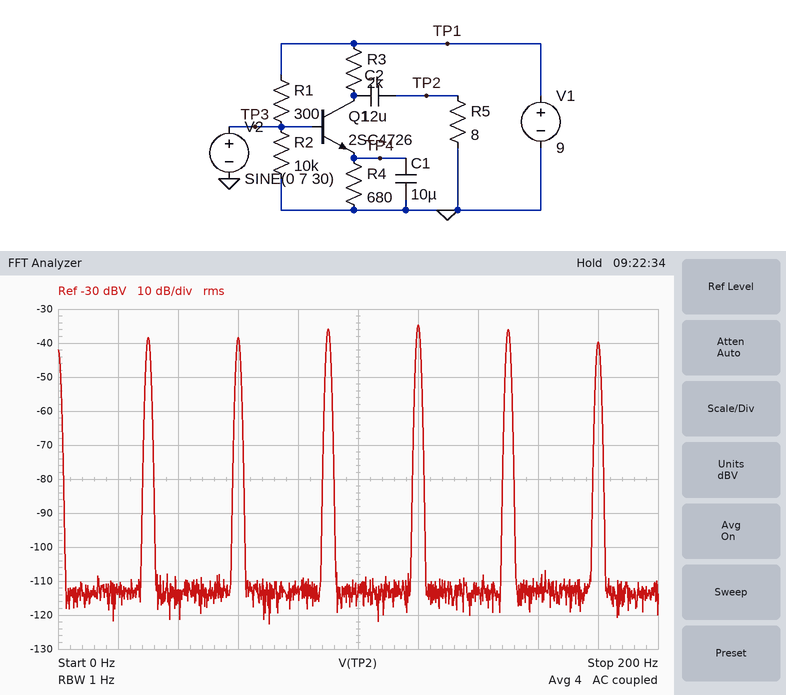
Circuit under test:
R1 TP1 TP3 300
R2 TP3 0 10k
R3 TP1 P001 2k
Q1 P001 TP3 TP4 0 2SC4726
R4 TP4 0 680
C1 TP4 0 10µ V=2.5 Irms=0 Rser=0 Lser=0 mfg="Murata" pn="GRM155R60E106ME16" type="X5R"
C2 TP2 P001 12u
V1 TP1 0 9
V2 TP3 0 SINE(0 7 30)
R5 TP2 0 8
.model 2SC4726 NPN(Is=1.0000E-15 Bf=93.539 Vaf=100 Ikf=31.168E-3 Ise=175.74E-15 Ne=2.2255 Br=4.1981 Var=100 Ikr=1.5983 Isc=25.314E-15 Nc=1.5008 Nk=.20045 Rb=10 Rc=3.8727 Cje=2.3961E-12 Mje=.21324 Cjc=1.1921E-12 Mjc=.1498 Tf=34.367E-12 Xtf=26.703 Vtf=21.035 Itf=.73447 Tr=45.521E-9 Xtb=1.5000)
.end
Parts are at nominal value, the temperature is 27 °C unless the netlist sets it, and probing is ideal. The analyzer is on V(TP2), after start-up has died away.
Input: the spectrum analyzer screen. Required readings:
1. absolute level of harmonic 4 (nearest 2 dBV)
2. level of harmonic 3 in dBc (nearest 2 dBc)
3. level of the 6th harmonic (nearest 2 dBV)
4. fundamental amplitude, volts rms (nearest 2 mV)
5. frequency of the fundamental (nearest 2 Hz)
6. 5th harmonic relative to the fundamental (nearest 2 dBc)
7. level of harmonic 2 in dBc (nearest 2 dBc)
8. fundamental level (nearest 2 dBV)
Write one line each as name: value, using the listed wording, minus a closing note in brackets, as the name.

absolute level of harmonic 4: -34 dBV
level of harmonic 3 in dBc: 2 dBc
level of the 6th harmonic: -40 dBV
fundamental amplitude, volts rms: 12 mV
frequency of the fundamental: 30 Hz
5th harmonic relative to the fundamental: 2 dBc
level of harmonic 2 in dBc: 0 dBc
fundamental level: -38 dBV
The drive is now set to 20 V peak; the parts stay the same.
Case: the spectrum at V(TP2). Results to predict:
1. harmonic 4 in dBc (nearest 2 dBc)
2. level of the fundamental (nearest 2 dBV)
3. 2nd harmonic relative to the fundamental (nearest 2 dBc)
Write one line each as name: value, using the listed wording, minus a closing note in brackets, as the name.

harmonic 4 in dBc: 2 dBc
level of the fundamental: -30 dBV
2nd harmonic relative to the fundamental: 2 dBc
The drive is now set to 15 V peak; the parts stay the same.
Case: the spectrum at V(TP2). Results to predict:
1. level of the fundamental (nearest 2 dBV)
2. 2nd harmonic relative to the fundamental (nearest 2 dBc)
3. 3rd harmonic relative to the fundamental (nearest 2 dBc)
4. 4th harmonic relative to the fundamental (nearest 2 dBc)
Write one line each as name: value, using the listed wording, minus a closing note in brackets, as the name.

level of the fundamental: -34 dBV
2nd harmonic relative to the fundamental: 4 dBc
3rd harmonic relative to the fundamental: 6 dBc
4th harmonic relative to the fundamental: 6 dBc
